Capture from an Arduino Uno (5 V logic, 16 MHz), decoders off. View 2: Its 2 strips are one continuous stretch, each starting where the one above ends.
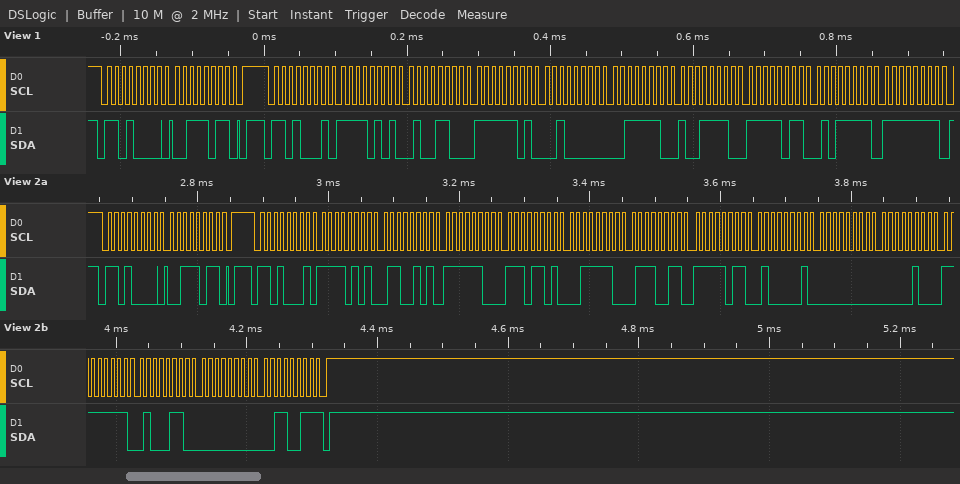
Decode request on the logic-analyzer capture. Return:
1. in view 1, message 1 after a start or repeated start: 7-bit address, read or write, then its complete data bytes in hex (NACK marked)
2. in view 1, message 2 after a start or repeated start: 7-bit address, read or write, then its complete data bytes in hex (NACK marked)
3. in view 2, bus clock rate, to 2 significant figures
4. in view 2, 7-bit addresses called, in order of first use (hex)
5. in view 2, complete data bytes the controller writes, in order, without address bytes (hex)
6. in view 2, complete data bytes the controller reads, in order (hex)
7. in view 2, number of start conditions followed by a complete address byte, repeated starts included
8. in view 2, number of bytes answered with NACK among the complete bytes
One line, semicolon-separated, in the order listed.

0x68 write: 3B; 0x68 read: F5 4C FD 20 3E 9E FB 5F FF; 100 kHz; 0x68; 3B; F5 65 FC ED 3E 73 FB 41 00 04 FF 46 00 33; 2; 1
